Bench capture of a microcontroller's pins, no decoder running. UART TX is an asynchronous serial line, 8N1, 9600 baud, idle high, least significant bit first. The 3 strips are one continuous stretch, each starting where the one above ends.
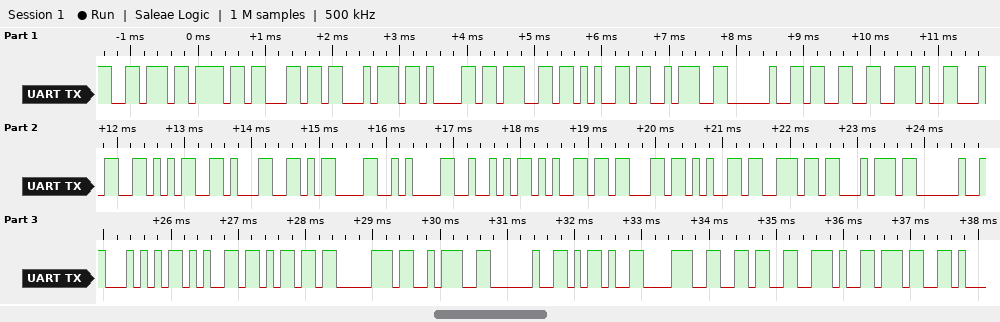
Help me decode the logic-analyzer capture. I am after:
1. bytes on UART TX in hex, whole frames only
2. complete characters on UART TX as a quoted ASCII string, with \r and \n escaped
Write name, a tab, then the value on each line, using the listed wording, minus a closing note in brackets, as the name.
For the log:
bytes on UART TX in hex, whole frames only	76 6F 6C 74 61 67 65 3A 20 33 2E 34 35 31 0D 0A 52 65 63 65 6E 74 20 54 65 6D 70 3A 20 2D 38 36 2E 37
complete characters on UART TX as a quoted ASCII string, with \r and \n escaped	"voltage: 3.451\r\nRecent Temp: -86.7"
